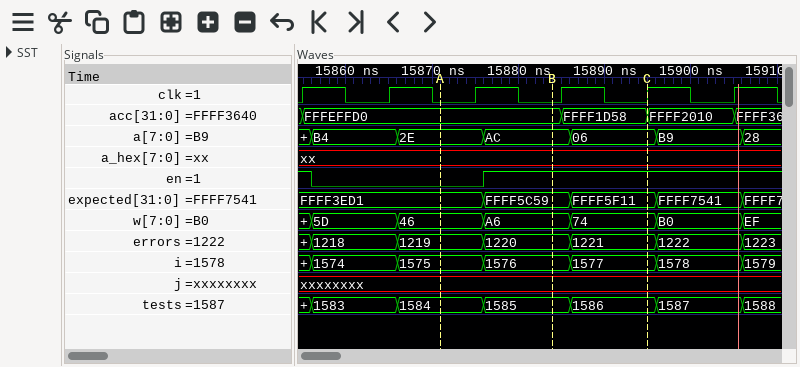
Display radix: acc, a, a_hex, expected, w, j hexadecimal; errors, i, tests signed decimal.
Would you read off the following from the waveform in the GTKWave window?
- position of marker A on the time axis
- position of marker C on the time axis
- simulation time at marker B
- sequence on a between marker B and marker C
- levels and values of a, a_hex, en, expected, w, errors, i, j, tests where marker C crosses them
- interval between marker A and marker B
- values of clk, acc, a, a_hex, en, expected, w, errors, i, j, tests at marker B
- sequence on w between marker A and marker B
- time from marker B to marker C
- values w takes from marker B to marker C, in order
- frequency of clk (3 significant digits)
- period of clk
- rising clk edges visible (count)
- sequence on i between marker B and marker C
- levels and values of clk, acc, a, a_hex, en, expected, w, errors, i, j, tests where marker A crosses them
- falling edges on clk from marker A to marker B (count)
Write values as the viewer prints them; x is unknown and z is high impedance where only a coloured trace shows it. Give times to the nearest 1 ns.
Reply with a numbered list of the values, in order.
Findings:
1. 15871 ns
2. 15895 ns
3. 15884 ns
4. AC, 06
5. a=06, a_hex=xx, en=1, expected=FFFF5F11, w=74, errors=1221, i=1577, j=xxxxxxxx, tests=1586
6. 13 ns
7. clk=0, acc=FFFEFFD0, a=AC, a_hex=xx, en=1, expected=FFFF5C59, w=A6, errors=1220, i=1576, j=xxxxxxxx, tests=1585
8. 46, A6
9. 11 ns
10. A6, 74
11. 100 MHz
12. 10 ns
13. 6
14. 1576, 1577
15. clk=0, acc=FFFEFFD0, a=2E, a_hex=xx, en=0, expected=FFFF3ED1, w=46, errors=1219, i=1575, j=xxxxxxxx, tests=1584
16. 1
